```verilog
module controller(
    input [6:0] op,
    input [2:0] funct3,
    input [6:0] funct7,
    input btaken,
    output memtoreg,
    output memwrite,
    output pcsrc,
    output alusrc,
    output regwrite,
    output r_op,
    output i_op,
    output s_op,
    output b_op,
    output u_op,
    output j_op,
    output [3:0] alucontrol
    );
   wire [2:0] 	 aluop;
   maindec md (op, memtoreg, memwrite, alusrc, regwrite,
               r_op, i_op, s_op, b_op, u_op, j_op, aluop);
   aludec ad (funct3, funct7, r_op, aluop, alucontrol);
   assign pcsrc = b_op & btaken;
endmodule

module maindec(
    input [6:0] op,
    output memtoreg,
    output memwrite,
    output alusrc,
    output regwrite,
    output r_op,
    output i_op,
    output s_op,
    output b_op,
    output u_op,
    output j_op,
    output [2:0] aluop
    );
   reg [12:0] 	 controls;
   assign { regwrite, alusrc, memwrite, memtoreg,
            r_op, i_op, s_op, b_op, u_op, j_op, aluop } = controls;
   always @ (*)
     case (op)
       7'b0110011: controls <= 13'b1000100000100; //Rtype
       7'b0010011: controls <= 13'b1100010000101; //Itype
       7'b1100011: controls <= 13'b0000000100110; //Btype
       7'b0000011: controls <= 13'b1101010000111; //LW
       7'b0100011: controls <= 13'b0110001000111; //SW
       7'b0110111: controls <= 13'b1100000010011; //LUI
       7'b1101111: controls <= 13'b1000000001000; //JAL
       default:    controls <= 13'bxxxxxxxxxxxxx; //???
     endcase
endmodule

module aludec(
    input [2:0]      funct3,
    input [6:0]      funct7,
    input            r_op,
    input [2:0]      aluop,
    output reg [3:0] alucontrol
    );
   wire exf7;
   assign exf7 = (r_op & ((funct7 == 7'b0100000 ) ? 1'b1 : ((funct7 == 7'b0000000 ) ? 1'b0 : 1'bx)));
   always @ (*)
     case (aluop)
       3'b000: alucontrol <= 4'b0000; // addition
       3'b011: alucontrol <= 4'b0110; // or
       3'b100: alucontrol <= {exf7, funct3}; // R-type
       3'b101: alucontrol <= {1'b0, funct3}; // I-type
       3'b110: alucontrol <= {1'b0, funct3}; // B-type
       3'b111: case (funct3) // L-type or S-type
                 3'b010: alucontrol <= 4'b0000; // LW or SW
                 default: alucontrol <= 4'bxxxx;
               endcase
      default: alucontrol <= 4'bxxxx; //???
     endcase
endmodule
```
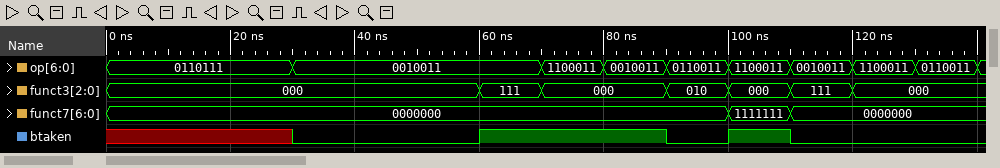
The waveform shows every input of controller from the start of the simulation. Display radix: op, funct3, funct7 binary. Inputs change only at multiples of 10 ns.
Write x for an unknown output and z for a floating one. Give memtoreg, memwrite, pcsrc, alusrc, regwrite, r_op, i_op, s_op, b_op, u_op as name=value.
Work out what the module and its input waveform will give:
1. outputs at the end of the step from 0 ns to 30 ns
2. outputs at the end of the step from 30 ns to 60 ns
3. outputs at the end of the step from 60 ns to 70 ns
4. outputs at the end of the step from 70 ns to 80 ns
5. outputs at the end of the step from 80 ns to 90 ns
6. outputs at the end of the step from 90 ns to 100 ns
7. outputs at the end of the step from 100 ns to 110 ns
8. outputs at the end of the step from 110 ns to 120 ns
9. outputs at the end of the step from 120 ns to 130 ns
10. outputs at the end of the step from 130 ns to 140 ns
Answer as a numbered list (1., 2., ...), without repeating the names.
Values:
1. memtoreg=0, memwrite=0, pcsrc=0, alusrc=1, regwrite=1, r_op=0, i_op=0, s_op=0, b_op=0, u_op=1
2. memtoreg=0, memwrite=0, pcsrc=0, alusrc=1, regwrite=1, r_op=0, i_op=1, s_op=0, b_op=0, u_op=0
3. memtoreg=0, memwrite=0, pcsrc=0, alusrc=1, regwrite=1, r_op=0, i_op=1, s_op=0, b_op=0, u_op=0
4. memtoreg=0, memwrite=0, pcsrc=1, alusrc=0, regwrite=0, r_op=0, i_op=0, s_op=0, b_op=1, u_op=0
5. memtoreg=0, memwrite=0, pcsrc=0, alusrc=1, regwrite=1, r_op=0, i_op=1, s_op=0, b_op=0, u_op=0
6. memtoreg=0, memwrite=0, pcsrc=0, alusrc=0, regwrite=1, r_op=1, i_op=0, s_op=0, b_op=0, u_op=0
7. memtoreg=0, memwrite=0, pcsrc=1, alusrc=0, regwrite=0, r_op=0, i_op=0, s_op=0, b_op=1, u_op=0
8. memtoreg=0, memwrite=0, pcsrc=0, alusrc=1, regwrite=1, r_op=0, i_op=1, s_op=0, b_op=0, u_op=0
9. memtoreg=0, memwrite=0, pcsrc=0, alusrc=0, regwrite=0, r_op=0, i_op=0, s_op=0, b_op=1, u_op=0
10. memtoreg=0, memwrite=0, pcsrc=0, alusrc=0, regwrite=1, r_op=1, i_op=0, s_op=0, b_op=0, u_op=0
